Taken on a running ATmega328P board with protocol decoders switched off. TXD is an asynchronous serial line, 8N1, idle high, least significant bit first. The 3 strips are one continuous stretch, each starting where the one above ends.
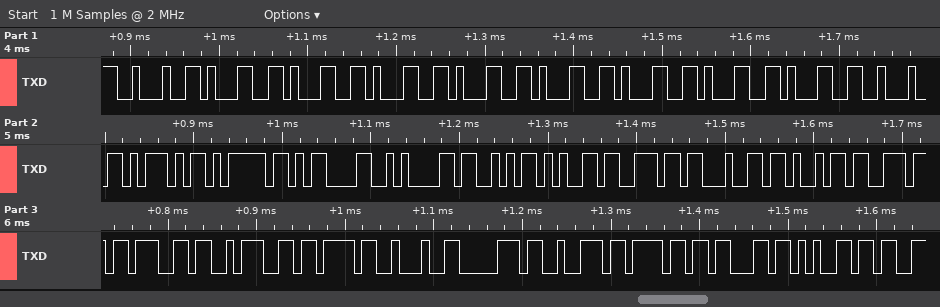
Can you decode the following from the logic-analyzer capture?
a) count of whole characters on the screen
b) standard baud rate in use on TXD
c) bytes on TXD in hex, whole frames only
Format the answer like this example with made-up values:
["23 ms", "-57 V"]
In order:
["29", "115200 baud", "0x22 0x31 0x31 0x31 0x31 0x31 0x31 0x31 0x31 0x22 0x5D 0x7D 0x0D 0x0A 0x53 0x65 0x6E 0x64 0x69 0x6E 0x67 0x3A 0x7B 0x22 0x70 0x72 0x6F 0x63 0x65"]
